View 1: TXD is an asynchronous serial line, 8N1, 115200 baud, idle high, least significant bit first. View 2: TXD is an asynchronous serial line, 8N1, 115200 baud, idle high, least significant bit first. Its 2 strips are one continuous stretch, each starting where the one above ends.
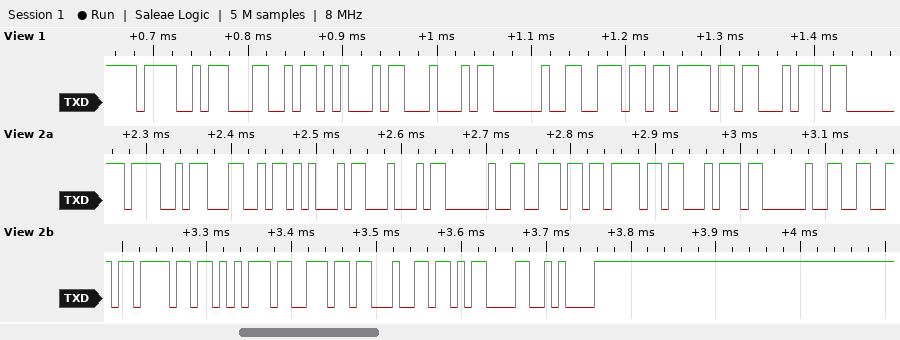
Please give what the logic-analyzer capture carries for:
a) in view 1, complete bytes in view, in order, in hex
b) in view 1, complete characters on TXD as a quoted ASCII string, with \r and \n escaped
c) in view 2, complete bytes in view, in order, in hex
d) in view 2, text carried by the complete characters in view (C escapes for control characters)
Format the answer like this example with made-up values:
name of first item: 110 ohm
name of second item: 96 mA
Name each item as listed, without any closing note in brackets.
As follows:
in view 1, complete bytes in view, in order, in hex: 4F 4C 45 44 20 6E 6F 74
in view 1, complete characters on TXD as a quoted ASCII string, with \r and \n escaped: "OLED not"
in view 2, complete bytes in view, in order, in hex: 4F 4C 45 44 20 6E 6F 74 20 66 6F 75 6E 64 0D 0A
in view 2, text carried by the complete characters in view: "OLED not found\r\n"
